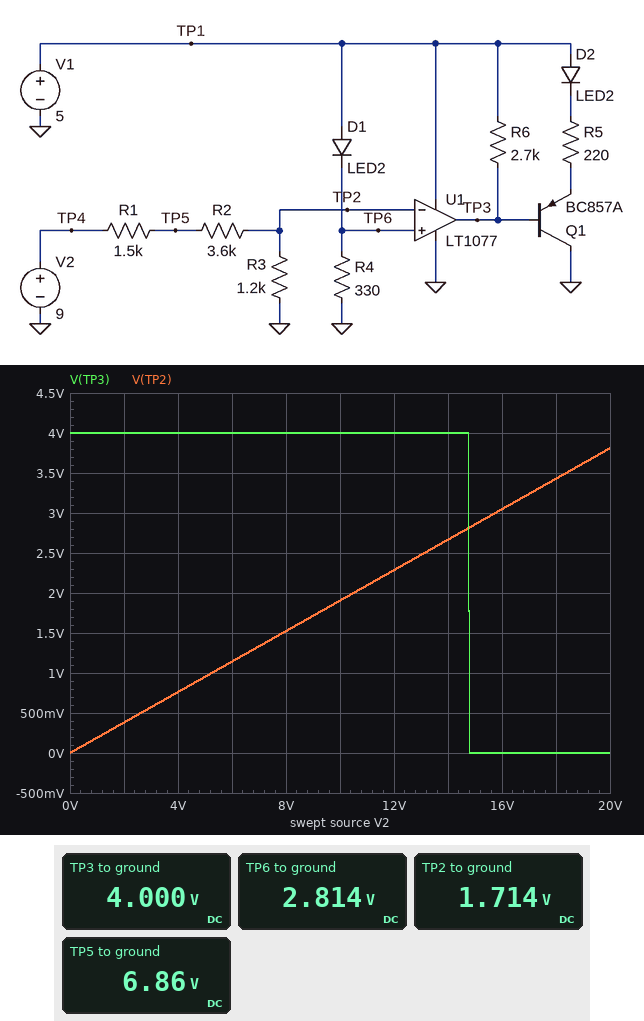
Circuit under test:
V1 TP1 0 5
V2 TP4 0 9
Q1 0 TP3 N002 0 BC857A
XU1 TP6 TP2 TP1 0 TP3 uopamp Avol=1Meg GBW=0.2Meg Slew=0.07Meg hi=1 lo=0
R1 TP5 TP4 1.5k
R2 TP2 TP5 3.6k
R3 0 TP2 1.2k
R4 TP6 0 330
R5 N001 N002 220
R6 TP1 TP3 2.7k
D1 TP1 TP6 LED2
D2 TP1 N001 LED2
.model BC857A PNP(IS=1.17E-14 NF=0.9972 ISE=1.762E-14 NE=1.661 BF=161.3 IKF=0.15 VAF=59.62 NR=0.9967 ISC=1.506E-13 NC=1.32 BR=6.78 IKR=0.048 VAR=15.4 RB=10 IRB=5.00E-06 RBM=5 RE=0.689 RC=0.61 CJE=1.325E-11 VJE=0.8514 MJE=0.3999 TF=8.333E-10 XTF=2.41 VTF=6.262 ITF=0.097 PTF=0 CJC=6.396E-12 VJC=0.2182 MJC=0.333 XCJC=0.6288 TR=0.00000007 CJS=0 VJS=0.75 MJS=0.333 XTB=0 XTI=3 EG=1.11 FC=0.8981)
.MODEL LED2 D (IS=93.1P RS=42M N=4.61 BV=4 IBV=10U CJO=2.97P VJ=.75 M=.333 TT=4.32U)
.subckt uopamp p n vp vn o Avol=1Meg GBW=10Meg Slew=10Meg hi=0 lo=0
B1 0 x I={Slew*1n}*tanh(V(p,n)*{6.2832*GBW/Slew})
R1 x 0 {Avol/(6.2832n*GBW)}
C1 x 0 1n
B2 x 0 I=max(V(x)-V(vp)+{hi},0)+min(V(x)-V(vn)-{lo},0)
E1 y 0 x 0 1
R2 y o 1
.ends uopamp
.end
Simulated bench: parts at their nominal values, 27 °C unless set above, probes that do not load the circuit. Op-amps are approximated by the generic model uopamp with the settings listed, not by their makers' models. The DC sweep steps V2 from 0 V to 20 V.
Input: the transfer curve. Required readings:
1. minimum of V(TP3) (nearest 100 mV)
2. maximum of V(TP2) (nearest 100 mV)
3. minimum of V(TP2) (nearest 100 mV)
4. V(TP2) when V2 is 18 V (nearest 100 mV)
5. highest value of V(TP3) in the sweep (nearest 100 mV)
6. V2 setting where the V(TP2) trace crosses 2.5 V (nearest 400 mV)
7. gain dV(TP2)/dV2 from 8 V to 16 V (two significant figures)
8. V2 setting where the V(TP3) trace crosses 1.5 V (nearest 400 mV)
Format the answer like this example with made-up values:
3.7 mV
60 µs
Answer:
0 V
3.8 V
0 V
3.4 V
4.0 V
13.2 V
0.19 V/V
14.8 V
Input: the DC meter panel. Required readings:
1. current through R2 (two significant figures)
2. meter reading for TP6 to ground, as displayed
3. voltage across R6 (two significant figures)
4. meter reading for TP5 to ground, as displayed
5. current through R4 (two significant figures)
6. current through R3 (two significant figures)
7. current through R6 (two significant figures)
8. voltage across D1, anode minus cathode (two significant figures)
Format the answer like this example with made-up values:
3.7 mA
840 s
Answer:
1.4 mA
2.814 V
1.0 V
6.86 V
8.5 mA
1.4 mA
370 µA
2.2 V
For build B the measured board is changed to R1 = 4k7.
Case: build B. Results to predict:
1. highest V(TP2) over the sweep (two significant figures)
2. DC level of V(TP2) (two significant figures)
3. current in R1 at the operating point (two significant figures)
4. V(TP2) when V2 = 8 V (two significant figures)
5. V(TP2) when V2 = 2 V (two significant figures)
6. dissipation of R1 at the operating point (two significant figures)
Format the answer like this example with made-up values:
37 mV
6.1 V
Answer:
2.5 V
1.1 V
950 µA
1.0 V
250 mV
4.2 mW
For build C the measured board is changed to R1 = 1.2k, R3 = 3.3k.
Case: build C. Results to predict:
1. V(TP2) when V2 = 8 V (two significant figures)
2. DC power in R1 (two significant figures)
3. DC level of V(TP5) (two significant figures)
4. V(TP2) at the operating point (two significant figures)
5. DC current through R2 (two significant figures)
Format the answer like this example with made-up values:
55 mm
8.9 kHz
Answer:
3.3 V
1.5 mW
7.7 V
3.7 V
1.1 mA
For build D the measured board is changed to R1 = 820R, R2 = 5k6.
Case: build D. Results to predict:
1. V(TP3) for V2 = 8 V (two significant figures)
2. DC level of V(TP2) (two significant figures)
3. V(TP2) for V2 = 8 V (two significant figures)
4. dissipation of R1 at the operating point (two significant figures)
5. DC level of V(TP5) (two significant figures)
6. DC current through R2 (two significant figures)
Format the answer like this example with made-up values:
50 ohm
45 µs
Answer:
4.0 V
1.4 V
1.3 V
1.1 mW
8.0 V
1.2 mA
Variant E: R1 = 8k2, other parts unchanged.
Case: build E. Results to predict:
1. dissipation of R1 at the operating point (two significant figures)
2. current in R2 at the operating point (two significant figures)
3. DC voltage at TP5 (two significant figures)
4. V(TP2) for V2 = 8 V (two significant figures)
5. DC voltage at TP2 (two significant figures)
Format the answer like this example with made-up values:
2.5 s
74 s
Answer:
3.9 mW
690 µA
3.3 V
740 mV
830 mV
